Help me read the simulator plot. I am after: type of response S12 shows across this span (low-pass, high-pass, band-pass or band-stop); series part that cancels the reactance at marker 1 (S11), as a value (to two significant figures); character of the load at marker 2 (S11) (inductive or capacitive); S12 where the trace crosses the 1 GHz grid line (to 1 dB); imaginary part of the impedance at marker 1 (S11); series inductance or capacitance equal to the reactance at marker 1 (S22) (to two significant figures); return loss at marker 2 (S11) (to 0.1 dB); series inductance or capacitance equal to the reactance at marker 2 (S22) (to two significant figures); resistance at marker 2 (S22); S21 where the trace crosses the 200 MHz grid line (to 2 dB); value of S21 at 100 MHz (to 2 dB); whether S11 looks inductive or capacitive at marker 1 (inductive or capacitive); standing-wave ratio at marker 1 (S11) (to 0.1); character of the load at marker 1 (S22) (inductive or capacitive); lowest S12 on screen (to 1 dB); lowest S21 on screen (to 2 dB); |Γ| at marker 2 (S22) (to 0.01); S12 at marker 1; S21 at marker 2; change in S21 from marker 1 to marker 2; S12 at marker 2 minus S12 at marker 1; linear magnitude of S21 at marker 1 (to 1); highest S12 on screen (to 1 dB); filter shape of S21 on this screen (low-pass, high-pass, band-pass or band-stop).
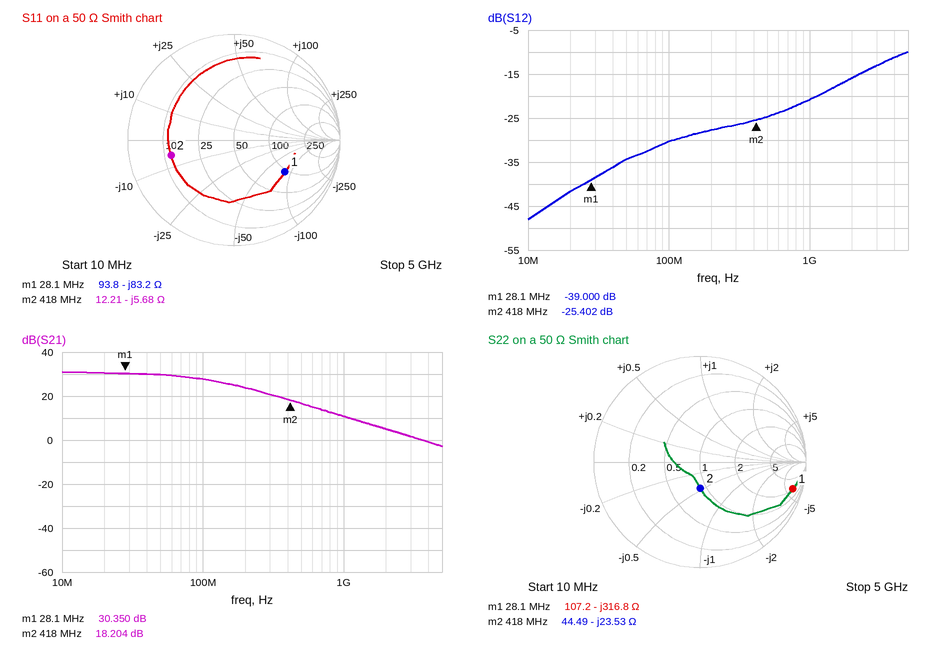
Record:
high-pass
470 nH
capacitive
-21 dB
-83.2 Ω
18 pF
4.3 dB
16 pF
44.49 Ω
24 dB
28 dB
capacitive
3.6
capacitive
-48 dB
-2 dB
0.25
-39.000 dB
18.204 dB
-12.146 dB
13.598 dB
33
-10 dB
low-pass
